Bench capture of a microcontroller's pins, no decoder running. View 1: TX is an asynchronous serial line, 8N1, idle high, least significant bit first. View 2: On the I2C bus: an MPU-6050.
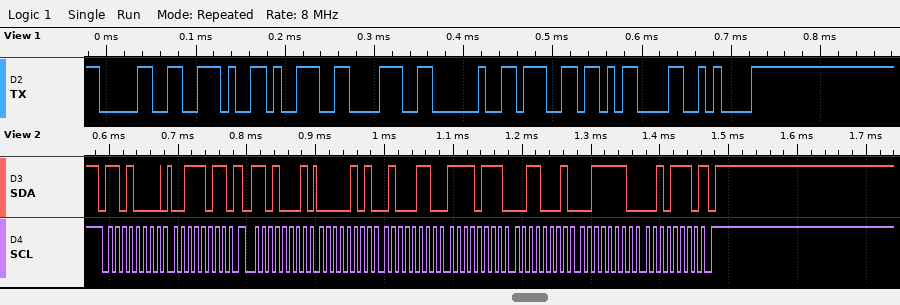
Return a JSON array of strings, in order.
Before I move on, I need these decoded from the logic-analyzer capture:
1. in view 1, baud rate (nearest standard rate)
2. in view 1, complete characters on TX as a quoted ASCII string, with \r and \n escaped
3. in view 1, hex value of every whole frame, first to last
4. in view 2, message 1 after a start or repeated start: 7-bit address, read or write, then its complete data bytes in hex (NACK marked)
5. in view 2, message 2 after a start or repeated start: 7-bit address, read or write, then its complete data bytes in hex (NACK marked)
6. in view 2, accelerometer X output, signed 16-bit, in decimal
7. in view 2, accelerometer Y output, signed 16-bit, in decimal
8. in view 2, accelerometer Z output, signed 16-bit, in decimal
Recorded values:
["115200 baud", "\"0.98 g\\r\\n\"", "0x30 0x2E 0x39 0x38 0x20 0x67 0x0D 0x0A", "0x68 write: 3B", "0x68 read: 05 46 F7 31 3E 2E NACK", "1350", "-2255", "15918"]
